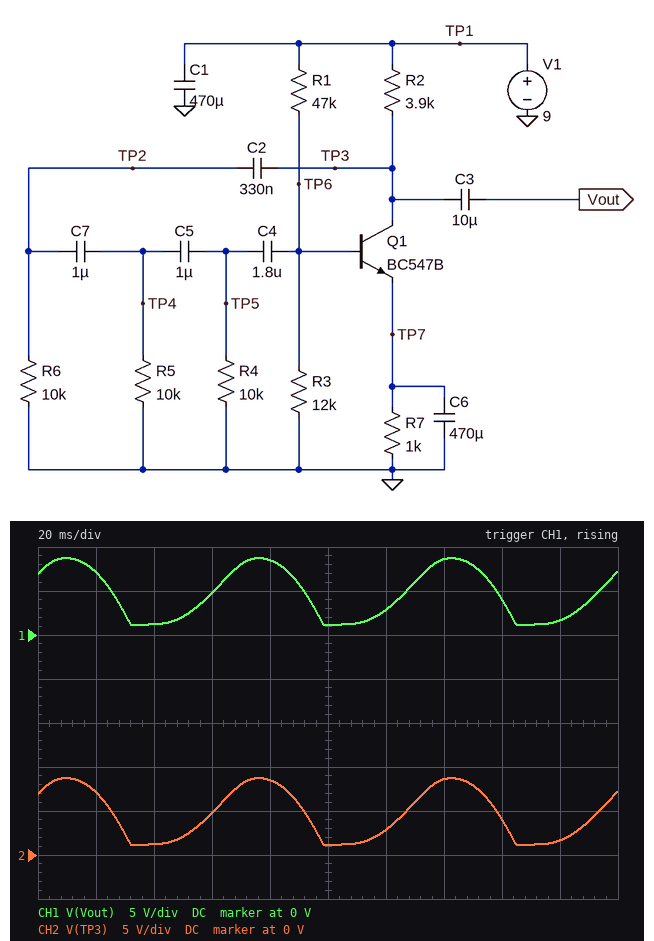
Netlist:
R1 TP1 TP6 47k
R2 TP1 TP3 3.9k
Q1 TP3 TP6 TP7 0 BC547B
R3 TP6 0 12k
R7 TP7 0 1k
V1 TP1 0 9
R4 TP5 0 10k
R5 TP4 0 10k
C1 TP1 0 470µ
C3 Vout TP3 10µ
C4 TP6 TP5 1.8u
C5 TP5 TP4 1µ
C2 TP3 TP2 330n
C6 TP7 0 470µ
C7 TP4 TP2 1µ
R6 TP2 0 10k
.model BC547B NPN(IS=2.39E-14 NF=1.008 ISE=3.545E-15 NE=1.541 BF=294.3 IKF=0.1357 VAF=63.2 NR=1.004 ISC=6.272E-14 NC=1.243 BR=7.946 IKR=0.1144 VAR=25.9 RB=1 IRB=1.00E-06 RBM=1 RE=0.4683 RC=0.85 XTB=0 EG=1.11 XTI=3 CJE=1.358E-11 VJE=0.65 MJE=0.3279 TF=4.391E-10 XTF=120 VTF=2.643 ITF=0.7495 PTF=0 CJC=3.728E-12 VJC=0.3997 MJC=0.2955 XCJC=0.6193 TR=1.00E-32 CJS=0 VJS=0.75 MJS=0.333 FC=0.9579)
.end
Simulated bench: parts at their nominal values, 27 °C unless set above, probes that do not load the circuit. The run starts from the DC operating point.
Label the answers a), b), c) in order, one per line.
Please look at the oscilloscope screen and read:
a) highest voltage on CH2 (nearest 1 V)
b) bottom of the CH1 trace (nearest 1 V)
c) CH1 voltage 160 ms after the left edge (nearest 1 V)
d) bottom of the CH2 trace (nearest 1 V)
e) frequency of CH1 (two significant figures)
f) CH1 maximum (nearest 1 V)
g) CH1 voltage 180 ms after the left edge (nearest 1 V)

a) 9 V
b) 1 V
c) 4 V
d) 1 V
e) 15 Hz
f) 9 V
g) 2 V
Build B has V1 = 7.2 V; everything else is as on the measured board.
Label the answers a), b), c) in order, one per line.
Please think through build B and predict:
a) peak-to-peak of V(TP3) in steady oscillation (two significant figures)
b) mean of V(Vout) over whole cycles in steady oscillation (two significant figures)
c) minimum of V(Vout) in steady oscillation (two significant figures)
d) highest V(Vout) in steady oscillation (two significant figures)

a) 6.3 V
b) 4.1 V
c) 850 mV
d) 7.1 V
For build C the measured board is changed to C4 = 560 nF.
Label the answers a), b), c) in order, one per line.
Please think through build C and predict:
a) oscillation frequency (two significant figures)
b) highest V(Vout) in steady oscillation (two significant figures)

a) 20 Hz
b) 8.6 V
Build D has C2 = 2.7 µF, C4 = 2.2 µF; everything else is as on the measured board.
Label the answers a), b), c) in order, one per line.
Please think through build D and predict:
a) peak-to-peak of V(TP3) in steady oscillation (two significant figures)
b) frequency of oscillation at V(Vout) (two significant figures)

a) 7.1 V
b) 8.7 Hz
